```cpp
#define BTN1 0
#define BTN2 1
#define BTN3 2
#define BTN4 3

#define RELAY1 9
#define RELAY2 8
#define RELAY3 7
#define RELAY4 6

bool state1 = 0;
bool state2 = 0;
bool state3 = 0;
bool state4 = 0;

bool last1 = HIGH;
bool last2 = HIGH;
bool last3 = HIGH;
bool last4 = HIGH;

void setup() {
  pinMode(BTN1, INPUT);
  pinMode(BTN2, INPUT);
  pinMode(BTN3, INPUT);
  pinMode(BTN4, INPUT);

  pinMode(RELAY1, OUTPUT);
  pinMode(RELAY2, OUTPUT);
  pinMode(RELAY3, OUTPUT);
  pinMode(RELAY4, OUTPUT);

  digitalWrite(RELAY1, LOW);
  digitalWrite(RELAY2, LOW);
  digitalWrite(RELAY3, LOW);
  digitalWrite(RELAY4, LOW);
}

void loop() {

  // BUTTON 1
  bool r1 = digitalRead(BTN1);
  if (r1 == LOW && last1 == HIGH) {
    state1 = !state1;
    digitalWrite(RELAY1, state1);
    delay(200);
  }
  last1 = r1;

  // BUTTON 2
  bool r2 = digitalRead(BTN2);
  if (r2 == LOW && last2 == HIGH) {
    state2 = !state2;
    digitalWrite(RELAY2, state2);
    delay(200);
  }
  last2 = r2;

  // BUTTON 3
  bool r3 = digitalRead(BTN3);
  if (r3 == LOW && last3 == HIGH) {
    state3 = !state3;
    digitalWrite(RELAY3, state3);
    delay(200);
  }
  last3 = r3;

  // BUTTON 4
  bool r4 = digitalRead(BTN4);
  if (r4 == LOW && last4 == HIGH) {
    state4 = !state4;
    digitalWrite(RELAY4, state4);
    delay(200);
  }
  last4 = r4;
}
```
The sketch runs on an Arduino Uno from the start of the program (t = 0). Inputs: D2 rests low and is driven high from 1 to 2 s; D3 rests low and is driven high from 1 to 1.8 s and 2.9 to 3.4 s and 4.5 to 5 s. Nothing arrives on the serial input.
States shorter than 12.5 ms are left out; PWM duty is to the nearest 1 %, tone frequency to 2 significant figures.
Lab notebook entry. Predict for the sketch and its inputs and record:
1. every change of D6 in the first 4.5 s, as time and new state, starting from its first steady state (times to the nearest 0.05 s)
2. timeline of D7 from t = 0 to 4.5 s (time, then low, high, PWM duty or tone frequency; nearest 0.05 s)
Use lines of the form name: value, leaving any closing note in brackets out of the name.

every change of D6 in the first 4.5 s, as time and new state, starting from its first steady state: 0 s low; 0.6 s high; 1.8 s low; 3.4 s high
timeline of D7 from t = 0 to 4.5 s: 0 s low; 0.4 s high; 2 s low
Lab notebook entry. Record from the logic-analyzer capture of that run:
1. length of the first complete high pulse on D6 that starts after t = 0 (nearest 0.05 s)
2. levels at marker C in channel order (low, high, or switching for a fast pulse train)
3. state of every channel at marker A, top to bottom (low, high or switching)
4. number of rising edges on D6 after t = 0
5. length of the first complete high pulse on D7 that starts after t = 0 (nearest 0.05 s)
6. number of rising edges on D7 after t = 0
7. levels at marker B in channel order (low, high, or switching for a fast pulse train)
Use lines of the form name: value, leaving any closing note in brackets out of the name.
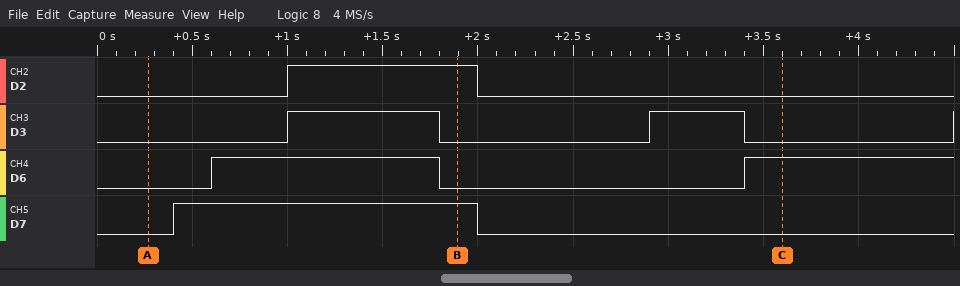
length of the first complete high pulse on D6 that starts after t = 0: 1.20 s
levels at marker C in channel order: D2 low, D3 low, D6 high, D7 low
state of every channel at marker A, top to bottom: D2 low, D3 low, D6 low, D7 low
number of rising edges on D6 after t = 0: 2
length of the first complete high pulse on D7 that starts after t = 0: 1.60 s
number of rising edges on D7 after t = 0: 1
levels at marker B in channel order: D2 high, D3 low, D6 low, D7 high
